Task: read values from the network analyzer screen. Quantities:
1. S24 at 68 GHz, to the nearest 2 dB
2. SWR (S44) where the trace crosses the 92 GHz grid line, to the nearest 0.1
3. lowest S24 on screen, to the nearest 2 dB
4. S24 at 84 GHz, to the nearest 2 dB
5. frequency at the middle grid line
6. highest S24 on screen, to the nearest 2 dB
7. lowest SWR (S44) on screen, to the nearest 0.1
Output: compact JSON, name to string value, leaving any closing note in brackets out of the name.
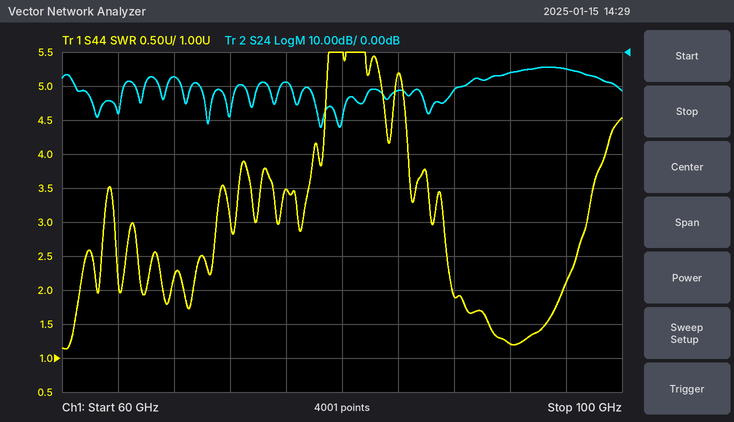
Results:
{"S24 at 68 GHz, to the nearest 2 dB": "-8 dB", "SWR (S44) where the trace crosses the 92 GHz grid line, to the nearest 0.1": "1.2", "lowest S24 on screen, to the nearest 2 dB": "-22 dB", "S24 at 84 GHz, to the nearest 2 dB": "-12 dB", "frequency at the middle grid line": "80 GHz", "highest S24 on screen, to the nearest 2 dB": "-4 dB", "lowest SWR (S44) on screen, to the nearest 0.1": "1.1"}
